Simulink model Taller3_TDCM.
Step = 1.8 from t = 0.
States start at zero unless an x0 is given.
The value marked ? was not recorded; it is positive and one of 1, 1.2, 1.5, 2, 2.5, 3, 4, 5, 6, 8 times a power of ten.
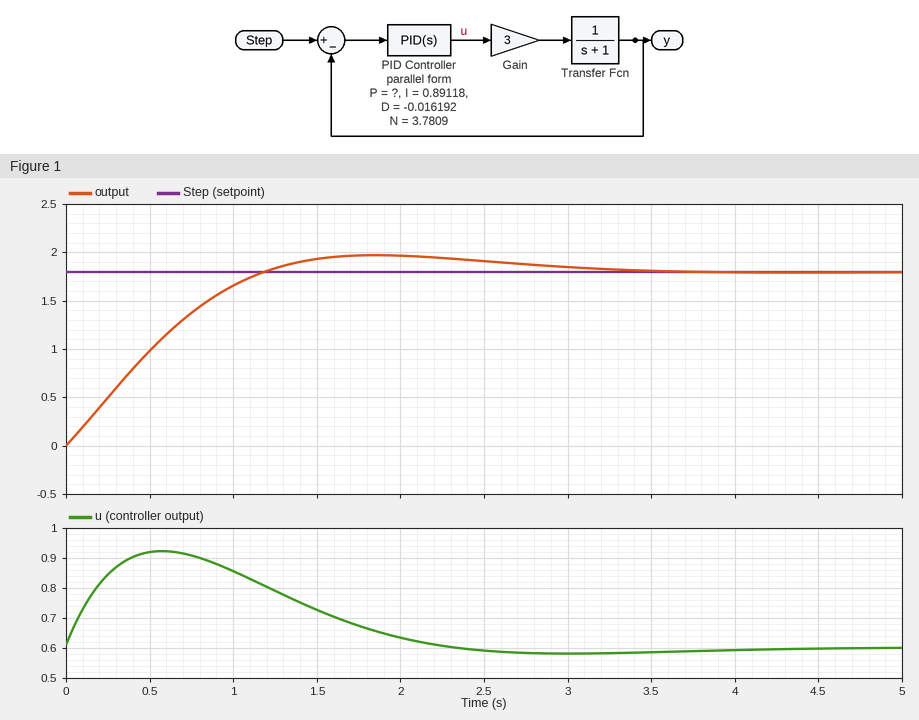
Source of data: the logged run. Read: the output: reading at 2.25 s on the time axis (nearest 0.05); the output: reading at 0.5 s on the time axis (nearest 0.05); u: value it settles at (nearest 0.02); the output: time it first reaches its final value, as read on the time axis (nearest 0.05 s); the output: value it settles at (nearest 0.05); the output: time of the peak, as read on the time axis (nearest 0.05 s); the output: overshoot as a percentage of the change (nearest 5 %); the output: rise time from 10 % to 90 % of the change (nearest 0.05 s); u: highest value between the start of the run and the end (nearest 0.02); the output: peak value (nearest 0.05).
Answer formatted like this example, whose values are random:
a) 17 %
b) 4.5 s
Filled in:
a) 1.95
b) 1.00
c) 0.60
d) 1.20 s
e) 1.80
f) 1.85 s
g) 10 %
h) 0.85 s
i) 0.92
j) 1.95
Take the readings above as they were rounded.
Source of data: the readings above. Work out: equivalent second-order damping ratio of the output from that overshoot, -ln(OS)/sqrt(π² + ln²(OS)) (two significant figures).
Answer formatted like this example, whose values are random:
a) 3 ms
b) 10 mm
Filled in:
a) 0.59
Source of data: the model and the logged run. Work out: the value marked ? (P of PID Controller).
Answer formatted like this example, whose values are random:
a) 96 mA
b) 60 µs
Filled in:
a) 0.4
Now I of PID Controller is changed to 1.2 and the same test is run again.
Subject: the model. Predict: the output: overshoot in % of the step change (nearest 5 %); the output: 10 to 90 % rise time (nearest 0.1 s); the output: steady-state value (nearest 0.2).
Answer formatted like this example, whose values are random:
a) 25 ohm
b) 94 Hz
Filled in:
a) 15 %
b) 0.7 s
c) 1.8
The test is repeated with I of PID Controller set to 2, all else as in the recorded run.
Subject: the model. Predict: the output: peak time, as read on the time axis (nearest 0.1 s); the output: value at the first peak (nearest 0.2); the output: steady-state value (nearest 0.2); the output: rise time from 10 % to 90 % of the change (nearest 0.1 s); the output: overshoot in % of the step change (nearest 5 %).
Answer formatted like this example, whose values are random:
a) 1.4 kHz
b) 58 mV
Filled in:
a) 1.2 s
b) 2.2
c) 1.8
d) 0.5 s
e) 25 %
